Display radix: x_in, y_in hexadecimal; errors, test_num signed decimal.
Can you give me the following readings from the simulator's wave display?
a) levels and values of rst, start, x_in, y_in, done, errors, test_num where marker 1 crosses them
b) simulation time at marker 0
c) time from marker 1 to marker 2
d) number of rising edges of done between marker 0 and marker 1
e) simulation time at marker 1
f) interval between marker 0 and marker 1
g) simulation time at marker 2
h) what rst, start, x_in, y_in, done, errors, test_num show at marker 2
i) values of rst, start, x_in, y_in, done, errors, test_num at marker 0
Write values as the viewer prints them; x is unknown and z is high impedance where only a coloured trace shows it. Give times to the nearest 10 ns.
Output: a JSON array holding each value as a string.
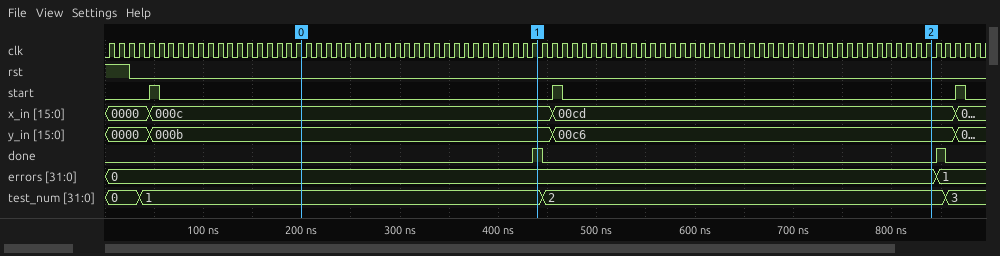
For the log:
["rst=0, start=0, x_in=000c, y_in=000b, done=1, errors=0, test_num=1", "200 ns", "400 ns", "1", "440 ns", "240 ns", "840 ns", "rst=0, start=0, x_in=00cd, y_in=00c6, done=0, errors=0, test_num=2", "rst=0, start=0, x_in=000c, y_in=000b, done=0, errors=0, test_num=1"]
